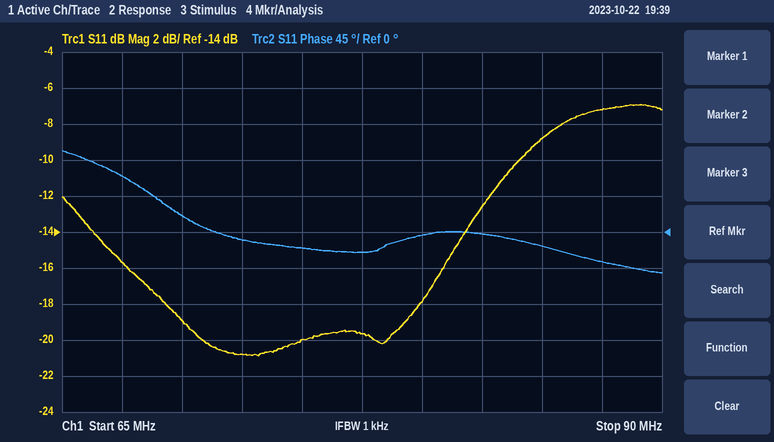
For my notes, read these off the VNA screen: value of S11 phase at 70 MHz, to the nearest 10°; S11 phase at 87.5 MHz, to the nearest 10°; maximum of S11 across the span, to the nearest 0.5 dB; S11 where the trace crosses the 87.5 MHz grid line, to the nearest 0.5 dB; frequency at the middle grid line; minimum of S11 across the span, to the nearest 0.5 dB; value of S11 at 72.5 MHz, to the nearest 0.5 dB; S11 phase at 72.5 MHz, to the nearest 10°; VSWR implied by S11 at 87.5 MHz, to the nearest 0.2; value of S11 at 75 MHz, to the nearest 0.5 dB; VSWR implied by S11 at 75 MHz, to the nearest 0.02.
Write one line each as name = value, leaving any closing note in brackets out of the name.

value of S11 phase at 70 MHz, to the nearest 10° = 20°
S11 phase at 87.5 MHz, to the nearest 10° = -40°
maximum of S11 across the span, to the nearest 0.5 dB = -7.0 dB
S11 where the trace crosses the 87.5 MHz grid line, to the nearest 0.5 dB = -7.0 dB
frequency at the middle grid line = 77.5 MHz
minimum of S11 across the span, to the nearest 0.5 dB = -21.0 dB
value of S11 at 72.5 MHz, to the nearest 0.5 dB = -21.0 dB
S11 phase at 72.5 MHz, to the nearest 10° = -10°
VSWR implied by S11 at 87.5 MHz, to the nearest 0.2 = 2.6
value of S11 at 75 MHz, to the nearest 0.5 dB = -20.0 dB
VSWR implied by S11 at 75 MHz, to the nearest 0.02 = 1.22
